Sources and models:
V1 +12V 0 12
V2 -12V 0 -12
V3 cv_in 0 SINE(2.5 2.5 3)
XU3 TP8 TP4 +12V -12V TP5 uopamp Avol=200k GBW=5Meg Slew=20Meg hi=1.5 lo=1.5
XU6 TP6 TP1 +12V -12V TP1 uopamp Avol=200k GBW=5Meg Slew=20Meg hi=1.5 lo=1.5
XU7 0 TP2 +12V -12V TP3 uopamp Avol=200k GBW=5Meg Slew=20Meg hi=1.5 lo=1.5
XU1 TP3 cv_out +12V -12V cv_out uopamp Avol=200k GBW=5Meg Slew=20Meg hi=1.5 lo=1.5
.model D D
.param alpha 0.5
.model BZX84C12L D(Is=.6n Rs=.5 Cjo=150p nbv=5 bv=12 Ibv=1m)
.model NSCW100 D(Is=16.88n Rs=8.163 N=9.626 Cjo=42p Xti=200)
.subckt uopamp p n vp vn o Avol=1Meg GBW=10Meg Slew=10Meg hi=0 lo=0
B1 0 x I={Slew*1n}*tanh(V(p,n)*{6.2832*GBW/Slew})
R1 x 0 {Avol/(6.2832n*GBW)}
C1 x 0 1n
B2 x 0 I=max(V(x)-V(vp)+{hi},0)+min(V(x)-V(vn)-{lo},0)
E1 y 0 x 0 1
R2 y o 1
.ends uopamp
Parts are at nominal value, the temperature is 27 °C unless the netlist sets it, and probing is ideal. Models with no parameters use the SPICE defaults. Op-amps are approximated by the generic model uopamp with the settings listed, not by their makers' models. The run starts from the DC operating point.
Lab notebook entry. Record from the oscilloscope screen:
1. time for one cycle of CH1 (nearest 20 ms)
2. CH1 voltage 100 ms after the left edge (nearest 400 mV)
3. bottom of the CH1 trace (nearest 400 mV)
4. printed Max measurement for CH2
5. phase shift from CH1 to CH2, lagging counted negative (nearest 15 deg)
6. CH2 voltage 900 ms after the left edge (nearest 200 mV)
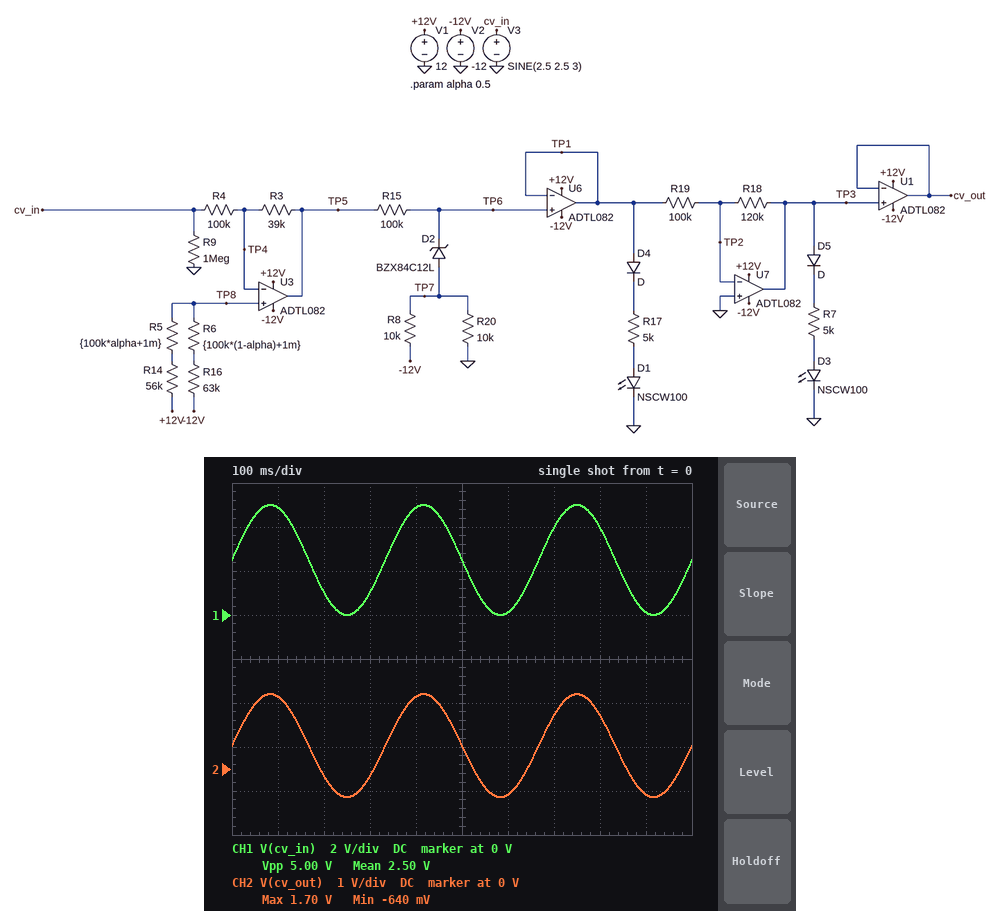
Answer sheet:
340 ms
4.8 V
0 V
1.70 V
0 deg
-600 mV
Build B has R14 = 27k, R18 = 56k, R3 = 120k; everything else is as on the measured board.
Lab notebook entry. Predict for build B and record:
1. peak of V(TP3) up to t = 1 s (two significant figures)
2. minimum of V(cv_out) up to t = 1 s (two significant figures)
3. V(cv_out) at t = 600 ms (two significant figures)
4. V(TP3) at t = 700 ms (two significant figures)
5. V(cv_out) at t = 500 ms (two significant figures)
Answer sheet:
560 mV
-2.8 V
-2.7 V
-130 mV
-1.1 V
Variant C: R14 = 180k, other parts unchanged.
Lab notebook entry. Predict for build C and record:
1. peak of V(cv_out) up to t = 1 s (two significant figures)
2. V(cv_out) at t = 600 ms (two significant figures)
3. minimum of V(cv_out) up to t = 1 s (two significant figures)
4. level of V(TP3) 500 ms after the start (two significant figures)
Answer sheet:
7.6 V
6.9 V
6.8 V
7.5 V
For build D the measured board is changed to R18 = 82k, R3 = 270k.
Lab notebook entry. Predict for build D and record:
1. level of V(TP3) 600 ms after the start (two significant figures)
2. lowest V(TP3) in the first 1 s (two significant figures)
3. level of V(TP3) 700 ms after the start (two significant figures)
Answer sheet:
-890 mV
-1.2 V
5.3 V
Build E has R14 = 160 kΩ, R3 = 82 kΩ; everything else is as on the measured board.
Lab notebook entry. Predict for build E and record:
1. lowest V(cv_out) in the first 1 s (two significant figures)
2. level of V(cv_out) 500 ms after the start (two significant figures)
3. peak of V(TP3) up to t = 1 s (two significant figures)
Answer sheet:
7.5 V
7.7 V
7.8 V
